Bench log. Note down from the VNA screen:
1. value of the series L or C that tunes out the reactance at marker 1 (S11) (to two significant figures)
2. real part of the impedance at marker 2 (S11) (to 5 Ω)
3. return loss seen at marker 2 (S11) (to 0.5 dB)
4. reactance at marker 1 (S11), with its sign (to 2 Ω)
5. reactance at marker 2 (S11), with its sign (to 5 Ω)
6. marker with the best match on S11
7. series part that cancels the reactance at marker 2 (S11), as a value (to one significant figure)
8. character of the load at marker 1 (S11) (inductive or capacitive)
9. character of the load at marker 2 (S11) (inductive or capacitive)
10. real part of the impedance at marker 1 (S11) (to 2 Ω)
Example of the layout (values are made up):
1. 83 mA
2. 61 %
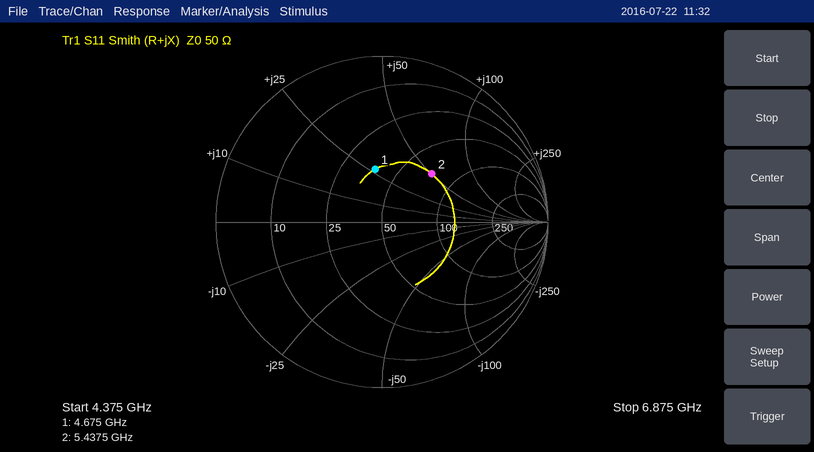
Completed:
1. 1.3 pF
2. 70 Ω
3. 7.5 dB
4. +26 Ω
5. +50 Ω
6. marker 1
7. 600 fF
8. inductive
9. inductive
10. 38 Ω
